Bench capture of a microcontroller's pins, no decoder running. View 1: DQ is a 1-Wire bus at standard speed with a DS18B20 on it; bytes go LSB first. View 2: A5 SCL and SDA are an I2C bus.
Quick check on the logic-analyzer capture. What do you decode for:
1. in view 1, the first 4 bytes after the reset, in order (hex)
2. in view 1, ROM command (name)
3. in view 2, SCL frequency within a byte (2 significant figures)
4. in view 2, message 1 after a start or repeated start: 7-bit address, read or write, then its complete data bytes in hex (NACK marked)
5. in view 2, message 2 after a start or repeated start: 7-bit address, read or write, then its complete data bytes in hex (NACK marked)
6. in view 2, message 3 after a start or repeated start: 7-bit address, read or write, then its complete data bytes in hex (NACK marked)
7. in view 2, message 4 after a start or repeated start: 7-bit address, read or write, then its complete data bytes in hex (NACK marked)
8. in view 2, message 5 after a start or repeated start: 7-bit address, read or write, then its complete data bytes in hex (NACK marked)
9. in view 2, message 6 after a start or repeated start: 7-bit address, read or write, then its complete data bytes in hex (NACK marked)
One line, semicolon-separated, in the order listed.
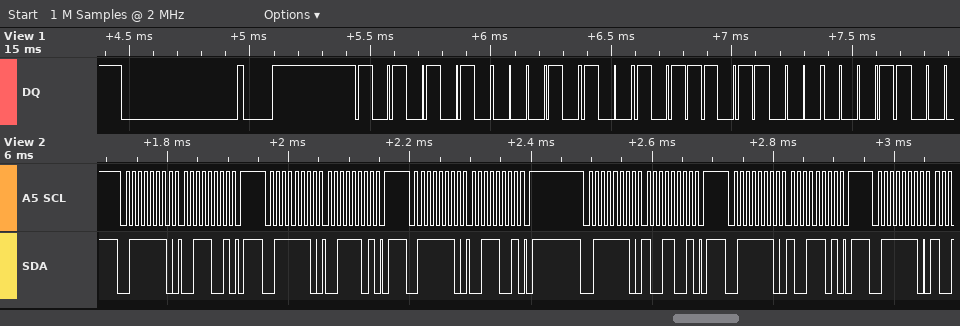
55 28 DD C0; Match ROM; 100 kHz; 0x3F write: 39; 0x3F write: 3D; 0x3F write: 39; 0x3F write: 99; 0x3F write: 9D; 0x3F write
